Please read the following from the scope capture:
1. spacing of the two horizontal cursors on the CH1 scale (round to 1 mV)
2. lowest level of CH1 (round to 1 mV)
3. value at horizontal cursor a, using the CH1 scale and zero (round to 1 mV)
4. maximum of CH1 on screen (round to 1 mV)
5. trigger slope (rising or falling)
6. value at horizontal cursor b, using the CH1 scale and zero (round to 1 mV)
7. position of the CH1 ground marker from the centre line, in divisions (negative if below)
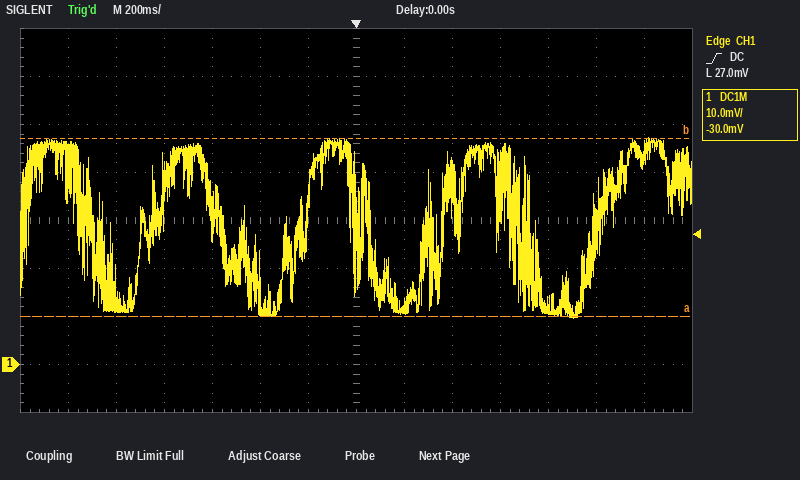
37 mV
10 mV
10 mV
47 mV
rising
47 mV
-3.0 div
